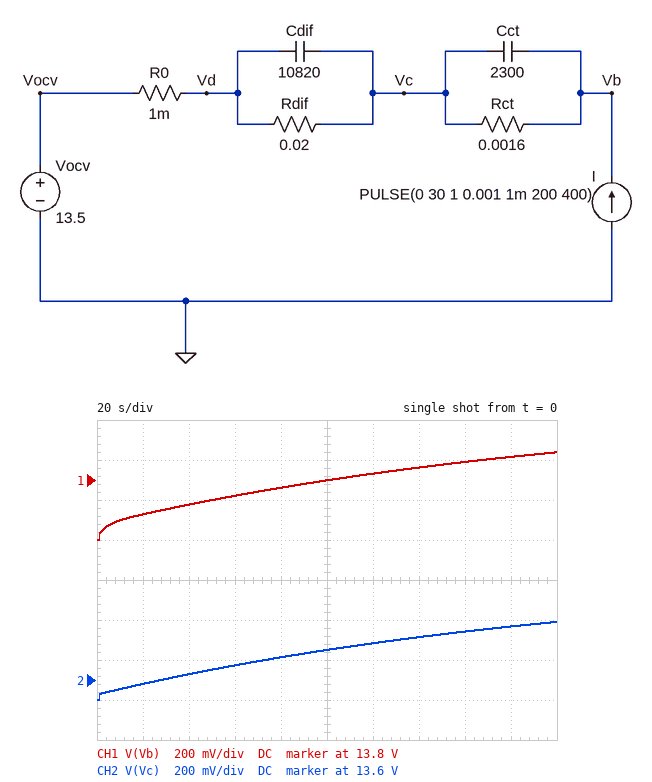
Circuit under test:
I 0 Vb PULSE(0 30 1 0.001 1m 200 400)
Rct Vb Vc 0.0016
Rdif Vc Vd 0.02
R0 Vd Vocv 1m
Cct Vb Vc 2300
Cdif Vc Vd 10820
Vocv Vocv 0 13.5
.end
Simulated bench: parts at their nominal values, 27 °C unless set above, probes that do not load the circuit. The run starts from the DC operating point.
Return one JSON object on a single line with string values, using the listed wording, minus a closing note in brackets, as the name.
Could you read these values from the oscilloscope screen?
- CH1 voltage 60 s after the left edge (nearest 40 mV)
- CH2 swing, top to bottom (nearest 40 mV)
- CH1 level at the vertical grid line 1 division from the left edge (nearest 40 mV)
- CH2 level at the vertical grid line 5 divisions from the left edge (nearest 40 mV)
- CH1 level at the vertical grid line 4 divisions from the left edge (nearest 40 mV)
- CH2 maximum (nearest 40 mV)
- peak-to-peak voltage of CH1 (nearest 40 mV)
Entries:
{"CH1 voltage 60 s after the left edge": "13.72 V", "CH2 swing, top to bottom": "400 mV", "CH1 level at the vertical grid line 1 division from the left edge": "13.64 V", "CH2 level at the vertical grid line 5 divisions from the left edge": "13.76 V", "CH1 level at the vertical grid line 4 divisions from the left edge": "13.76 V", "CH2 maximum": "13.88 V", "peak-to-peak voltage of CH1": "440 mV"}
